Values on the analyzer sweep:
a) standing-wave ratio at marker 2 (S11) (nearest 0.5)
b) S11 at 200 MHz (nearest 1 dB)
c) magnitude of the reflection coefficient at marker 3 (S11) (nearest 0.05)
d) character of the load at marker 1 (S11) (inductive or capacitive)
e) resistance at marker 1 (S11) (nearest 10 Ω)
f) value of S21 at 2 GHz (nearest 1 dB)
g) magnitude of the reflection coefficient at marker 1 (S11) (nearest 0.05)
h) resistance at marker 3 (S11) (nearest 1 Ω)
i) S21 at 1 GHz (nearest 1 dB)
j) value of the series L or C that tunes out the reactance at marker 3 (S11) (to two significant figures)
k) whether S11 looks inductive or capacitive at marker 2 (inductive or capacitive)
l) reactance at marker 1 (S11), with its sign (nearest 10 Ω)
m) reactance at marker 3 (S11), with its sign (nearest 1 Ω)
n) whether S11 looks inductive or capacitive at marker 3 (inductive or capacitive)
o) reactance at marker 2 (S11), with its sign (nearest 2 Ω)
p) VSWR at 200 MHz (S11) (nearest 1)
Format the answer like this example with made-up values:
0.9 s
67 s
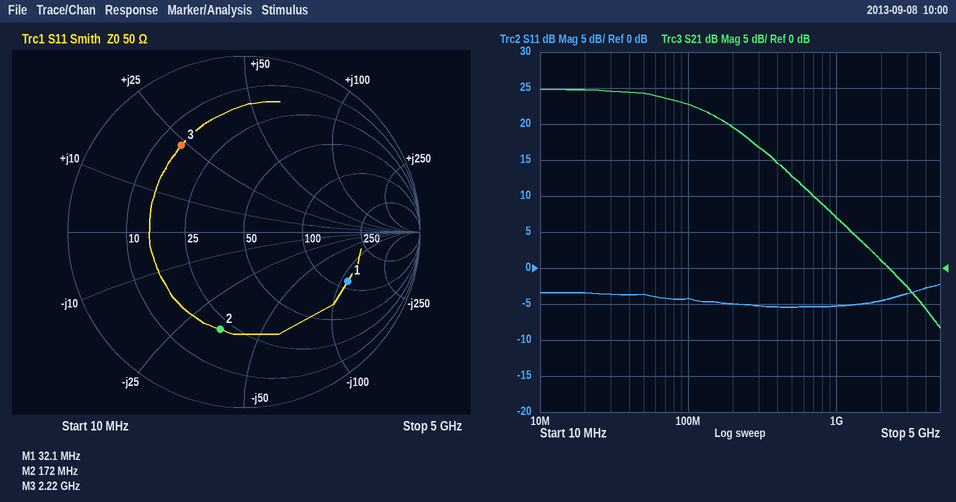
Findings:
3.5
-5 dB
0.60
capacitive
120 Ω
1 dB
0.65
15 Ω
7 dB
3.0 pF
capacitive
-110 Ω
+24 Ω
inductive
-34 Ω
4
